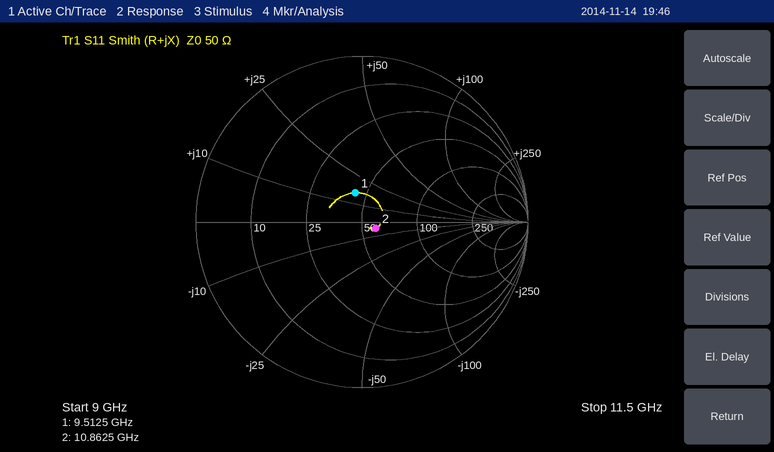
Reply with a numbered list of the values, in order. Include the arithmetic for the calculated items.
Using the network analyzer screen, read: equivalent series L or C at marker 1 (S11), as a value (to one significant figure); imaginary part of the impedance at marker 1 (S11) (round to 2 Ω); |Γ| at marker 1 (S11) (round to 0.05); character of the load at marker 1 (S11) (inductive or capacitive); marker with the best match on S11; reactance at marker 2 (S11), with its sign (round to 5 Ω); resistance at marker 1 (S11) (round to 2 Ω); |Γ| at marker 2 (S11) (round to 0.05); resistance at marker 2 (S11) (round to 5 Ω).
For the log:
1. L = 16 Ω/(2π × 9.5125 GHz) ≈ 268 pH, so 300 pH to one significant figure
2. +16 Ω
3. 0.20
4. inductive
5. marker 2
6. -5 Ω
7. 44 Ω
8. 0.10
9. 60 Ω
